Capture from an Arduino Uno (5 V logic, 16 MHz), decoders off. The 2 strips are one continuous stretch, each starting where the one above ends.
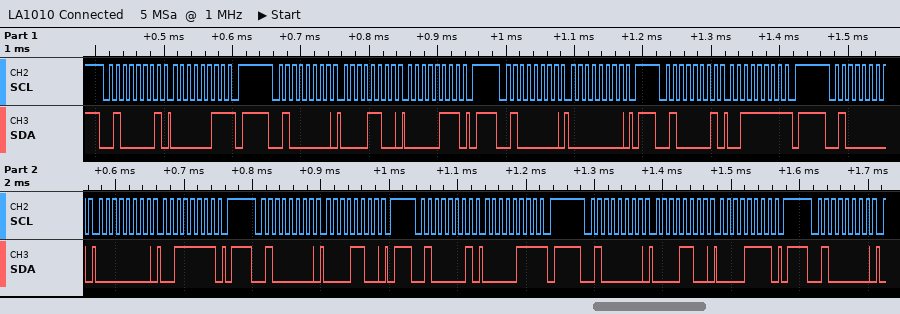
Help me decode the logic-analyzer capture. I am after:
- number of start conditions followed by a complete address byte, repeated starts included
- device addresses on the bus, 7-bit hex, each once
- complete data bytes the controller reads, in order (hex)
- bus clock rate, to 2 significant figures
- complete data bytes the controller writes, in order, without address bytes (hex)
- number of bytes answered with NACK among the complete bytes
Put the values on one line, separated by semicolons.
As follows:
9; 0x20; 03 3F 07; 100 kHz; 0C 07 00 00 3F 0C 0C 0F; 3
